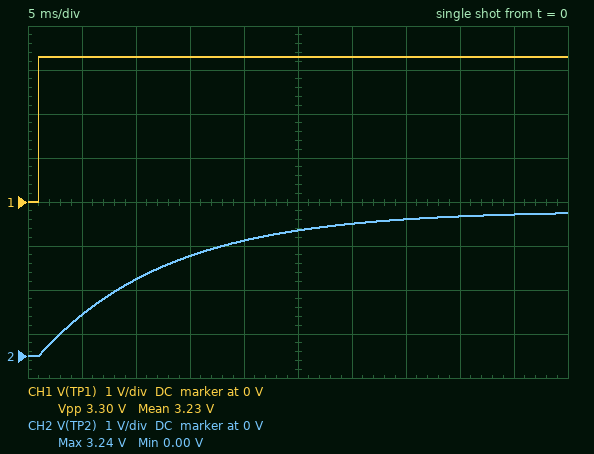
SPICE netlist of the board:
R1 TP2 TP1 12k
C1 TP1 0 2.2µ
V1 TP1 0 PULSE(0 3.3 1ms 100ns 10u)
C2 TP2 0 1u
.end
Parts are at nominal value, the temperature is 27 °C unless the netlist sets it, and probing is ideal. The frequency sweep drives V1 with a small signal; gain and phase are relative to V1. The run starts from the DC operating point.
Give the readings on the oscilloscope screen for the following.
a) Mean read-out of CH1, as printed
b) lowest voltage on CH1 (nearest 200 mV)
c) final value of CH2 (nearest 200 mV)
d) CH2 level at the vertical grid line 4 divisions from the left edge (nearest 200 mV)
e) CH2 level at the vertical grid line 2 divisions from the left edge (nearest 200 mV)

3.23 V
0 V
3.2 V
2.6 V
1.8 V
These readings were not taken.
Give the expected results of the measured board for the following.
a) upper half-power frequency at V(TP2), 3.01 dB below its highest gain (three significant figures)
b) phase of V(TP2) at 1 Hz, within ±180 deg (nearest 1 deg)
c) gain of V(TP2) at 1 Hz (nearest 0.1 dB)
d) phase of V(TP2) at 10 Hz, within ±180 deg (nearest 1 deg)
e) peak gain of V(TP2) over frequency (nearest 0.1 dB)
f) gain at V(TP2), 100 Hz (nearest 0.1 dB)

13.3 Hz
-4 deg
0 dB
-37 deg
0 dB
-17.6 dB
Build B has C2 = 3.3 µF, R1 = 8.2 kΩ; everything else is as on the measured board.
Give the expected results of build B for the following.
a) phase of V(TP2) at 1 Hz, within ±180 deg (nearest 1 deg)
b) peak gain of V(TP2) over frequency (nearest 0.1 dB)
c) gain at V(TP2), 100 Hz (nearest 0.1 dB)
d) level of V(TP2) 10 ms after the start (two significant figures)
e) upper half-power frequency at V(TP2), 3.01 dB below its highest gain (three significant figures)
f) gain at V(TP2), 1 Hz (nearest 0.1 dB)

-10 deg
0 dB
-24.6 dB
930 mV
5.88 Hz
-0.1 dB
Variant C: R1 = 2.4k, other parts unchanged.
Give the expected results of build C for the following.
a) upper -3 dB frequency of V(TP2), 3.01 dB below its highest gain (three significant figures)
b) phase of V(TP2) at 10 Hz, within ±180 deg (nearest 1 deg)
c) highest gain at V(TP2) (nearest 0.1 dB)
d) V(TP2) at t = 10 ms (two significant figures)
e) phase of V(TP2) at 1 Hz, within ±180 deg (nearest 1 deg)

66.3 Hz
-9 deg
0 dB
3.2 V
-1 deg
